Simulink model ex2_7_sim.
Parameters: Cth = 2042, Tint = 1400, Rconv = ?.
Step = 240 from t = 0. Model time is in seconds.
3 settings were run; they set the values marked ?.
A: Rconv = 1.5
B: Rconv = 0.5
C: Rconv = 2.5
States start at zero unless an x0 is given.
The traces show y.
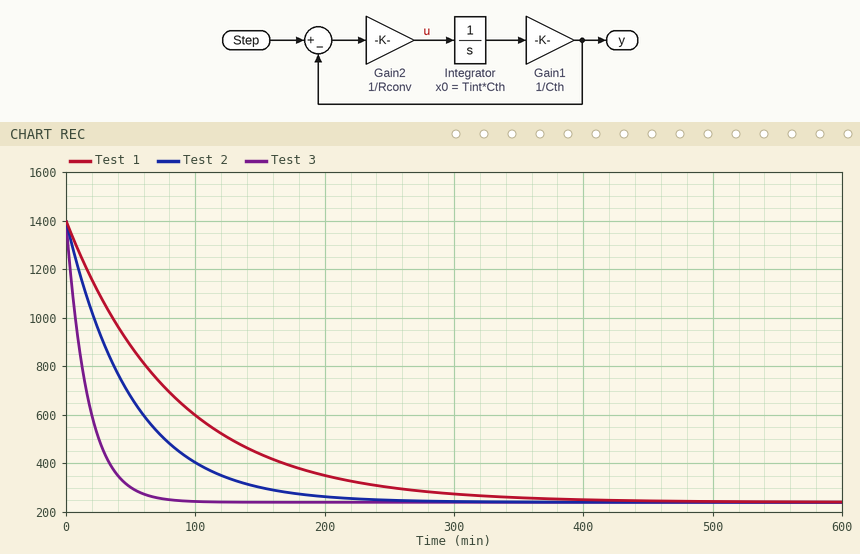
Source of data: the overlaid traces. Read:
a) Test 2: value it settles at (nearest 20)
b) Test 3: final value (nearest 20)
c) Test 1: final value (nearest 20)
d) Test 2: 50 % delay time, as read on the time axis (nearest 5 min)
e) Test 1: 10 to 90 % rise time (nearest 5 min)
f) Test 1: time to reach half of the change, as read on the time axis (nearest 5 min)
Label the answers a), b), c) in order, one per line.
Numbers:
a) 240
b) 240
c) 240
d) 35 min
e) 185 min
f) 60 min
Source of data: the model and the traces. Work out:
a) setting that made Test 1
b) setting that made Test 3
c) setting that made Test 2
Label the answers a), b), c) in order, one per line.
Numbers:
a) C
b) B
c) A
